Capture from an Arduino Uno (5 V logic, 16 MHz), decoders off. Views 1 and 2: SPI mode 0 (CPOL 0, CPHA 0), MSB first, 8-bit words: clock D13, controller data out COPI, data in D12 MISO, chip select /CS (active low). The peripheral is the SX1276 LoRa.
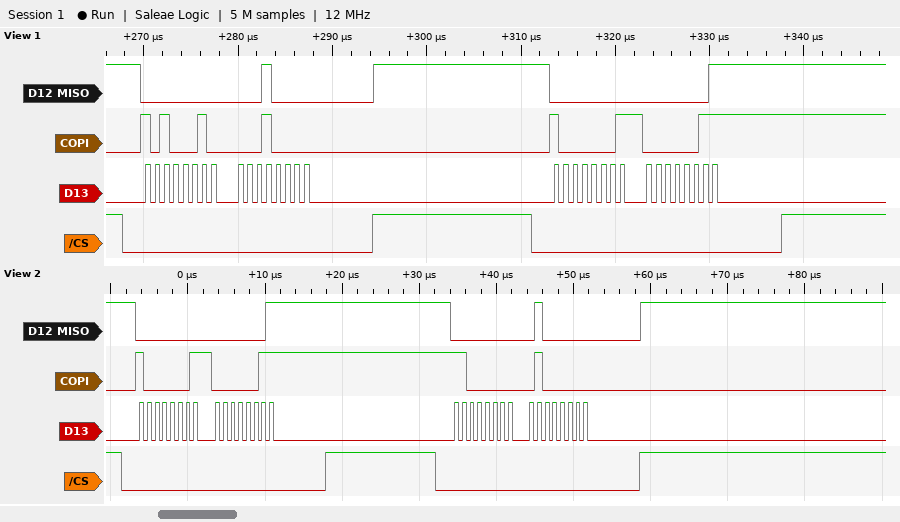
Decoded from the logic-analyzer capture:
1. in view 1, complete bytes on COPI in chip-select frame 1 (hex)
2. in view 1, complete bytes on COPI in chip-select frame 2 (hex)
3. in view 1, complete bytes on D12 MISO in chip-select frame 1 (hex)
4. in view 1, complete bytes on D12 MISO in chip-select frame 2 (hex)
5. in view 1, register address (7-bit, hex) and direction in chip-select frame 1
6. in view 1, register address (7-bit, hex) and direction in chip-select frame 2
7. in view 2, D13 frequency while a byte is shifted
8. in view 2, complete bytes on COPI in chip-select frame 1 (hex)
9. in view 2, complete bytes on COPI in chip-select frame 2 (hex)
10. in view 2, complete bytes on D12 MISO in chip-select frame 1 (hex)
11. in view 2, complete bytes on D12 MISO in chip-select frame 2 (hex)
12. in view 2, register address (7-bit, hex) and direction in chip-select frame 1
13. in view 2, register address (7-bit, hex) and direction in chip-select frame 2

0xA2 0x10
0x81 0x03
0x00 0x10
0x00 0x01
0x22 write
0x01 write
1 MHz
81 03
C0 40
00 01
00 40
0x01 write
0x40 write
